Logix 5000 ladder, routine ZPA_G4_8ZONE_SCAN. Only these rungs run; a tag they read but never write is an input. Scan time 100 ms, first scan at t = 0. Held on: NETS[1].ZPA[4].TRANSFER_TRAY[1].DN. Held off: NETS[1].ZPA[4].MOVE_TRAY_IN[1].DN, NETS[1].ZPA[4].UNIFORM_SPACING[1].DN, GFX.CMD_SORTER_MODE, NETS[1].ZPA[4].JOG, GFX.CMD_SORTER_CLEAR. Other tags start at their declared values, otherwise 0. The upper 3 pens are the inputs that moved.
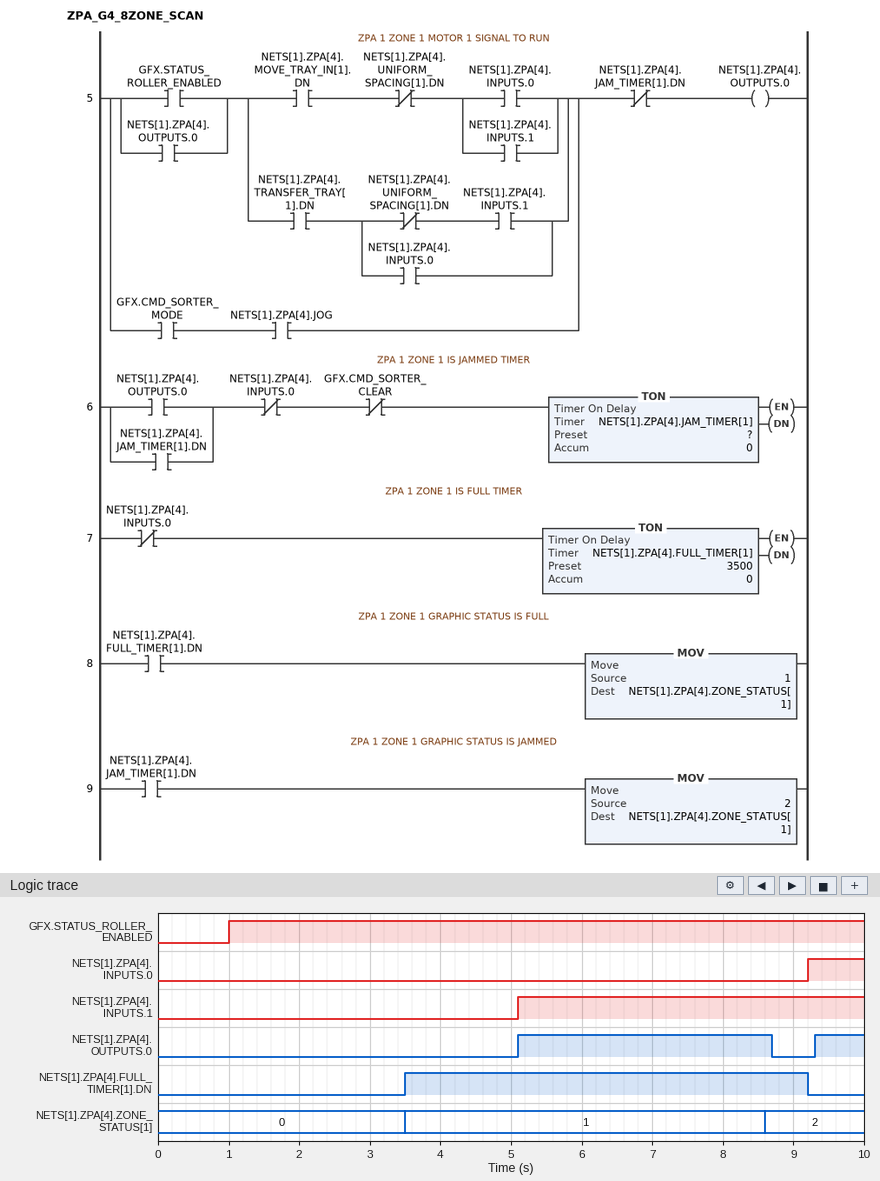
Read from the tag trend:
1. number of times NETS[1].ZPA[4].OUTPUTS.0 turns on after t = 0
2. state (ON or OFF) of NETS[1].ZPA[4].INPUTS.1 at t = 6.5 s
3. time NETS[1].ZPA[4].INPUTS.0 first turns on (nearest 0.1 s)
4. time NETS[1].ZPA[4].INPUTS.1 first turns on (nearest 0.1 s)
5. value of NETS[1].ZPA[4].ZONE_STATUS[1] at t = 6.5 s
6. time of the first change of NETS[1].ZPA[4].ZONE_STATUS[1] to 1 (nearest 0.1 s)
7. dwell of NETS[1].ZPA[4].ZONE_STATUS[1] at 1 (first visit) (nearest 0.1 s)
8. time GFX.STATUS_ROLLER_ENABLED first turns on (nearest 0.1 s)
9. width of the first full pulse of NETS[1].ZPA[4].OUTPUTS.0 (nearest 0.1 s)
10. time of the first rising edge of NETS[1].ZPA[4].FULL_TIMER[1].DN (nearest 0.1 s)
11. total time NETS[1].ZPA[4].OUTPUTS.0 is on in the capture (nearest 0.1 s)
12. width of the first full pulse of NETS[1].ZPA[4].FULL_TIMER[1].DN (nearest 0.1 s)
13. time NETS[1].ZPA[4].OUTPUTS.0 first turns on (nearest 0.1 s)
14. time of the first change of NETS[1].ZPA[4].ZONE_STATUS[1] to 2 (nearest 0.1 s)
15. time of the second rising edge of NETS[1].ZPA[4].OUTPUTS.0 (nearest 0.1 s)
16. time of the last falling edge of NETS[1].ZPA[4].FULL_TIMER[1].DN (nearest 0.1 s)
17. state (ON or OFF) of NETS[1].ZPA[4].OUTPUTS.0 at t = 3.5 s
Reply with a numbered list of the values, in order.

1. 2
2. ON
3. 9.2 s
4. 5.1 s
5. 1
6. 3.5 s
7. 5.1 s
8. 1.0 s
9. 3.6 s
10. 3.5 s
11. 4.3 s
12. 5.7 s
13. 5.1 s
14. 8.6 s
15. 9.3 s
16. 9.2 s
17. OFF
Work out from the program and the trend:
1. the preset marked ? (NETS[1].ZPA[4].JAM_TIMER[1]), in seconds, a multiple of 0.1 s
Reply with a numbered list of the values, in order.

1. 3.5 s
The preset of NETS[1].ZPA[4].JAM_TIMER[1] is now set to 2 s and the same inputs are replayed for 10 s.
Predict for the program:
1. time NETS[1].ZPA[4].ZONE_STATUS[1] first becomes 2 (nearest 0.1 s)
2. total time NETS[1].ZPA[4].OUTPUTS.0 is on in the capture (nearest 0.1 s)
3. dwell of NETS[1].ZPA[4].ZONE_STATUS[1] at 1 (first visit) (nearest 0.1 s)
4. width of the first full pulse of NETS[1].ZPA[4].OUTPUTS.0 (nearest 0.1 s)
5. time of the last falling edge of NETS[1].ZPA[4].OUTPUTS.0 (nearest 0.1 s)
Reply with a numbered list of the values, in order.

1. 7.1 s
2. 2.8 s
3. 3.6 s
4. 2.1 s
5. 7.2 s
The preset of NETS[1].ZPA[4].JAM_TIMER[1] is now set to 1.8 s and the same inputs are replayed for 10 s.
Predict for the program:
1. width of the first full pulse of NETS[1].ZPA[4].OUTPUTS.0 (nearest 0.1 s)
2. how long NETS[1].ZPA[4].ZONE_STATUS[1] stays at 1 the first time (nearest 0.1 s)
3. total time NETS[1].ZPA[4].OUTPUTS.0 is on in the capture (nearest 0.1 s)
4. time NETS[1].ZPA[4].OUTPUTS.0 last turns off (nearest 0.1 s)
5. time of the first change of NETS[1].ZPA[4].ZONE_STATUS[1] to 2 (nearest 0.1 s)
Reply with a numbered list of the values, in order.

1. 1.9 s
2. 3.4 s
3. 2.6 s
4. 7.0 s
5. 6.9 s
